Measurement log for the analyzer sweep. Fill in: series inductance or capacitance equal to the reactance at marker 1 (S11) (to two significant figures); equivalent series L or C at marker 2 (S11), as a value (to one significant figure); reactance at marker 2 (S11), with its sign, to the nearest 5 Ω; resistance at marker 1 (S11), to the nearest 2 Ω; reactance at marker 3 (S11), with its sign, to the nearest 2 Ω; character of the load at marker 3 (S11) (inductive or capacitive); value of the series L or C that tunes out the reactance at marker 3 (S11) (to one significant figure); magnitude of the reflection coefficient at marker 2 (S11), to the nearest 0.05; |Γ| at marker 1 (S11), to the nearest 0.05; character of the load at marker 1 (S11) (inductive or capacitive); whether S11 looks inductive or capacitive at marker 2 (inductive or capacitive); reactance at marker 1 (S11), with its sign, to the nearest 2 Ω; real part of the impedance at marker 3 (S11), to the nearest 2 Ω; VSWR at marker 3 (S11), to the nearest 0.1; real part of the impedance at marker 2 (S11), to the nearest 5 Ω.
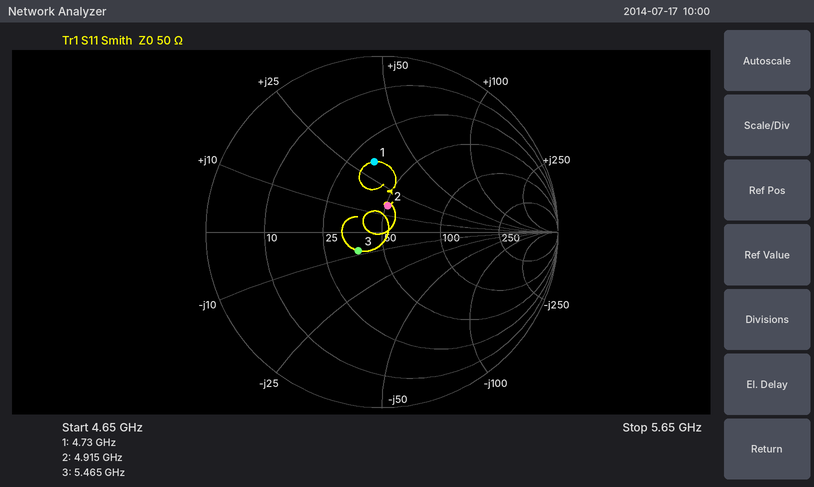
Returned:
1.1 nH
500 pH
+15 Ω
34 Ω
-8 Ω
capacitive
200 pH
0.15
0.40
inductive
inductive
+32 Ω
38 Ω
1.4
50 Ω
